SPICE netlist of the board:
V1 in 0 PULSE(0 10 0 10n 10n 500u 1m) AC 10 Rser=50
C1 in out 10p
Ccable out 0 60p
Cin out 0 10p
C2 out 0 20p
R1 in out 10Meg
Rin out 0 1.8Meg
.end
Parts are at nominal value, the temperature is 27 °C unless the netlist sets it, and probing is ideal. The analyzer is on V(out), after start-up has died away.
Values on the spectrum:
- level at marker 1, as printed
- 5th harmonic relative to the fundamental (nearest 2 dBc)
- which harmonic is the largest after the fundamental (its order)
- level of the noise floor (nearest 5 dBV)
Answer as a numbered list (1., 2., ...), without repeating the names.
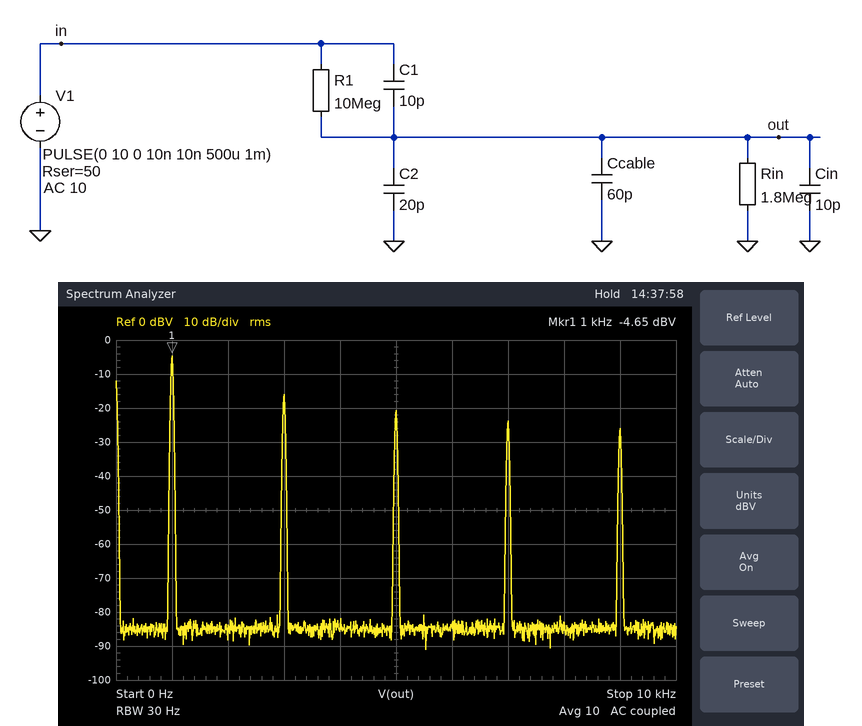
1. -4.65 dBV
2. -16 dBc
3. 3
4. -85 dBV
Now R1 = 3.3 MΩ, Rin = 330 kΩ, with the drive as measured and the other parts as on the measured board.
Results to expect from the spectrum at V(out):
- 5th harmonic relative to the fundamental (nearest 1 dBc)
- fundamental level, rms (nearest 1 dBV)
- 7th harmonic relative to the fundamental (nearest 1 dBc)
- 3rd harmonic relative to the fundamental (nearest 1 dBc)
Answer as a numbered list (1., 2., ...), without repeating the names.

1. -14 dBc
2. -8 dBV
3. -16 dBc
4. -9 dBc
